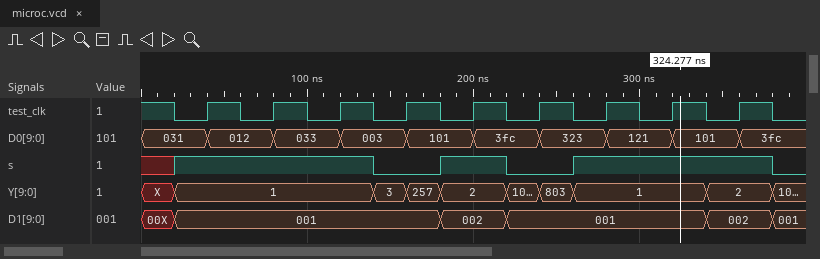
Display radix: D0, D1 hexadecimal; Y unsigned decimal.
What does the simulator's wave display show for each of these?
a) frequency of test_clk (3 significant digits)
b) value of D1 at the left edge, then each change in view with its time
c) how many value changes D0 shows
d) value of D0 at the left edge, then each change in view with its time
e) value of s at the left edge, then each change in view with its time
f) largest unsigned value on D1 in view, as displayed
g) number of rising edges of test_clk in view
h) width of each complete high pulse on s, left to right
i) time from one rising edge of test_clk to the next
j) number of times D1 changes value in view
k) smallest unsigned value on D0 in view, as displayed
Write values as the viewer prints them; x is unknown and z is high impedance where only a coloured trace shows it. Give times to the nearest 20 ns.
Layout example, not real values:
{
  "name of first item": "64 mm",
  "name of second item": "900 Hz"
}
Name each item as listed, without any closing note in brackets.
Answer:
{
  "frequency of test_clk": "25.0 MHz",
  "value of D1 at the left edge, then each change in view with its time": "00X, 001 at 20 ns, 002 at 180 ns, 001 at 220 ns, 002 at 340 ns, 001 at 380 ns",
  "how many value changes D0 shows": "9",
  "value of D0 at the left edge, then each change in view with its time": "031, 012 at 40 ns, 033 at 80 ns, 003 at 120 ns, 101 at 160 ns, 3fc at 200 ns, 323 at 240 ns, 121 at 280 ns, 101 at 320 ns, 3fc at 360 ns",
  "value of s at the left edge, then each change in view with its time": "x, 1 at 20 ns, 0 at 140 ns, 1 at 180 ns, 0 at 220 ns, 1 at 260 ns, 0 at 380 ns",
  "largest unsigned value on D1 in view, as displayed": "002",
  "number of rising edges of test_clk in view": "9",
  "width of each complete high pulse on s, left to right": "40 ns, 120 ns",
  "time from one rising edge of test_clk to the next": "40 ns",
  "number of times D1 changes value in view": "5",
  "smallest unsigned value on D0 in view, as displayed": "003"
}
